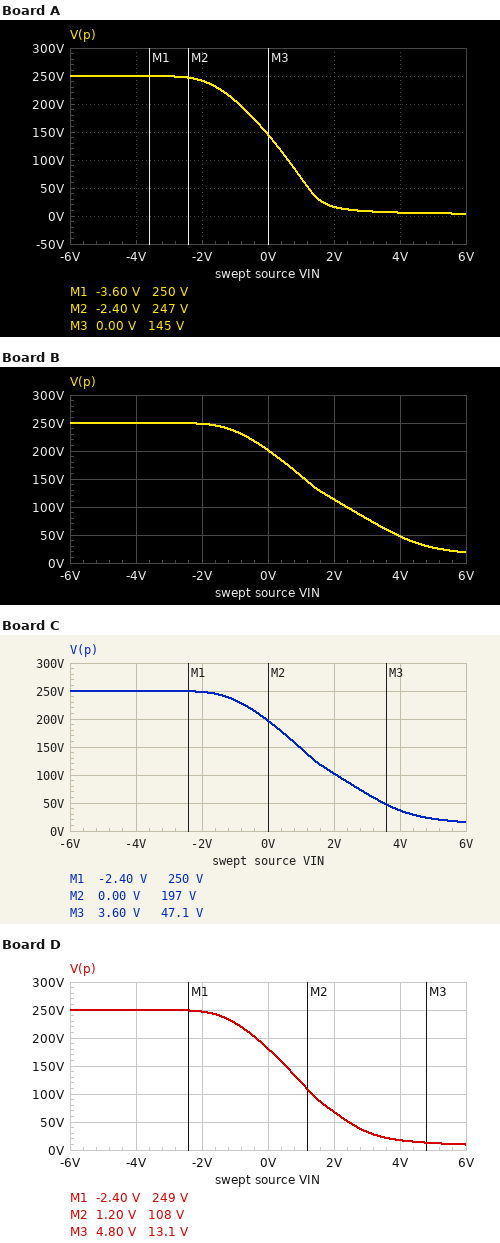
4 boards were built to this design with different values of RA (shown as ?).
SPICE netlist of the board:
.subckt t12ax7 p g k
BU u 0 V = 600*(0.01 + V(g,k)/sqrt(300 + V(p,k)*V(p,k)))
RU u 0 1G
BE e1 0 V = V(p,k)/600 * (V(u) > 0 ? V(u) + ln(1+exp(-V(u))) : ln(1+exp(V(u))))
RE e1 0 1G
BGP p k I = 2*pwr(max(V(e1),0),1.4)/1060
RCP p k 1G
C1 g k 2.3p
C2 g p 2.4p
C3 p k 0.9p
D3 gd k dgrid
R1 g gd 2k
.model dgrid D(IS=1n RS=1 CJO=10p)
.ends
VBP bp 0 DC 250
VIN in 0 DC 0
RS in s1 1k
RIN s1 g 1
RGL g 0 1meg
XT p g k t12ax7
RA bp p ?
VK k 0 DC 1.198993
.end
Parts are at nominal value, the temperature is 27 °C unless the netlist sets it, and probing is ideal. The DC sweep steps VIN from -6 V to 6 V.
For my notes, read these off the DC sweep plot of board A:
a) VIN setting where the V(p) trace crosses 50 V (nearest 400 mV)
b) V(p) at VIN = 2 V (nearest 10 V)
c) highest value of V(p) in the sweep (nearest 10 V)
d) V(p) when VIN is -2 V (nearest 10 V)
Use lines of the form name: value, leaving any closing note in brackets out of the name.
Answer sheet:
VIN setting where the V(p) trace crosses 50 V: 1.2 V
V(p) at VIN = 2 V: 20 V
highest value of V(p) in the sweep: 250 V
V(p) when VIN is -2 V: 240 V
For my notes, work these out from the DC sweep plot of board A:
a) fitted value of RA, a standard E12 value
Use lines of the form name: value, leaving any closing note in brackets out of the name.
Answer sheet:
fitted value of RA, a standard E12 value: 270 kΩ
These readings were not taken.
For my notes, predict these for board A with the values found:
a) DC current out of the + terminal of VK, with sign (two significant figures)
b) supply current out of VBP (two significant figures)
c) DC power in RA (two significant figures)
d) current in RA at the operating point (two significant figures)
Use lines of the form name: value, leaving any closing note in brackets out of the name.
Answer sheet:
DC current out of the + terminal of VK, with sign: -390 µA
supply current out of VBP: 390 µA
DC power in RA: 41 mW
current in RA at the operating point: 390 µA
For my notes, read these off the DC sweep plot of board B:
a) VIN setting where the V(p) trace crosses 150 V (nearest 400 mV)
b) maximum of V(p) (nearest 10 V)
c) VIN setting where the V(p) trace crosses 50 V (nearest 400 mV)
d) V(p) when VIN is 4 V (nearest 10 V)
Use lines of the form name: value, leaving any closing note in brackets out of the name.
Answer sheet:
VIN setting where the V(p) trace crosses 150 V: 1.2 V
maximum of V(p): 250 V
VIN setting where the V(p) trace crosses 50 V: 4.0 V
V(p) when VIN is 4 V: 50 V
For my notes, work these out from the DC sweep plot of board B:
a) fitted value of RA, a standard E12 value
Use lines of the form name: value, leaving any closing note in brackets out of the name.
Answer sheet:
fitted value of RA, a standard E12 value: 33 kΩ
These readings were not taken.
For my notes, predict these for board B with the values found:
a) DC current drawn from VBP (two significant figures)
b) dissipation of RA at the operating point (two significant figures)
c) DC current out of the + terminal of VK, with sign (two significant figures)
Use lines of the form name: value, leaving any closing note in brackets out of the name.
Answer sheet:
DC current drawn from VBP: 1.5 mA
dissipation of RA at the operating point: 71 mW
DC current out of the + terminal of VK, with sign: -1.5 mA
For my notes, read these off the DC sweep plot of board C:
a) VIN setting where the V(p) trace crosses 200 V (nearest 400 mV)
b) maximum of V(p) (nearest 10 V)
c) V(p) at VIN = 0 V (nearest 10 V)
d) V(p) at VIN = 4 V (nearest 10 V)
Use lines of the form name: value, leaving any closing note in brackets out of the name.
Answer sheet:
VIN setting where the V(p) trace crosses 200 V: 0 V
maximum of V(p): 250 V
V(p) at VIN = 0 V: 200 V
V(p) at VIN = 4 V: 40 V
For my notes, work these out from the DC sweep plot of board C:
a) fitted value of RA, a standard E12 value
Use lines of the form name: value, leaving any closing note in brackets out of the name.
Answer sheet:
fitted value of RA, a standard E12 value: 39 kΩ
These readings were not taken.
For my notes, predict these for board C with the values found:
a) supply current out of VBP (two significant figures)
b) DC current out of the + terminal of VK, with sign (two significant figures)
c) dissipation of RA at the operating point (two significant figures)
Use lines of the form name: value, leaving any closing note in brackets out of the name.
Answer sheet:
supply current out of VBP: 1.4 mA
DC current out of the + terminal of VK, with sign: -1.4 mA
dissipation of RA at the operating point: 72 mW
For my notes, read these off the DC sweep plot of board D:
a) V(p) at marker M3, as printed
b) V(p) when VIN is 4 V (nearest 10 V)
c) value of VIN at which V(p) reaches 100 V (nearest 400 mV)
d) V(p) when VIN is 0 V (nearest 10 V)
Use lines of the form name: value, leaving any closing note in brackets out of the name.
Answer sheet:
V(p) at marker M3, as printed: 13.1 V
V(p) when VIN is 4 V: 20 V
value of VIN at which V(p) reaches 100 V: 1.2 V
V(p) when VIN is 0 V: 180 V
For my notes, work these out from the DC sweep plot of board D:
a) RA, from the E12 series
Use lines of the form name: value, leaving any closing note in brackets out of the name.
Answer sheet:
RA, from the E12 series: 68 kΩ
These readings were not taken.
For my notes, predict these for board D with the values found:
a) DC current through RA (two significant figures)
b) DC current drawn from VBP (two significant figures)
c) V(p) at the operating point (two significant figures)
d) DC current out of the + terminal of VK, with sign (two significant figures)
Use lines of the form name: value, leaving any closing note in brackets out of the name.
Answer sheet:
DC current through RA: 1.0 mA
DC current drawn from VBP: 1.0 mA
V(p) at the operating point: 180 V
DC current out of the + terminal of VK, with sign: -1.0 mA
